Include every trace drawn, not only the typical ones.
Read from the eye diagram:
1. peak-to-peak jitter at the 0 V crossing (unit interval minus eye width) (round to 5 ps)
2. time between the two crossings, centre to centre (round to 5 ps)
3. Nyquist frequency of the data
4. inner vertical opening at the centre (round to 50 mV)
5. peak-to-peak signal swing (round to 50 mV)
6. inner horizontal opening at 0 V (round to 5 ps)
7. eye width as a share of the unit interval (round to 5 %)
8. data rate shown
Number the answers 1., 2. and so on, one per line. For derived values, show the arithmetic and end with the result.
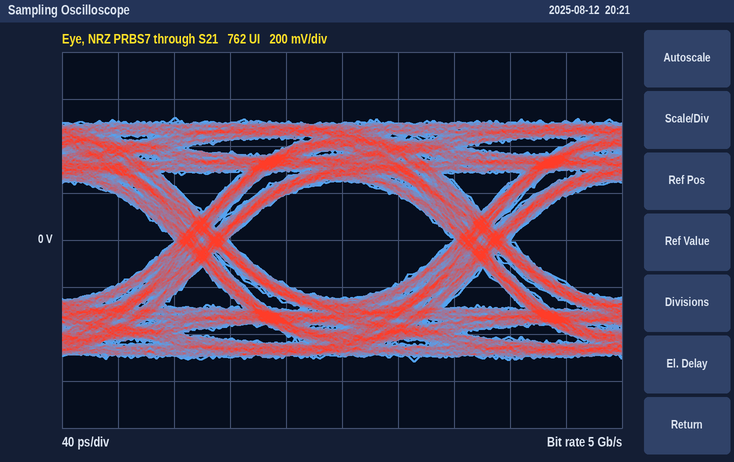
1. 40 ps
2. 200 ps
3. 2.5 GHz
4. 500 mV
5. 1.05 V
6. 160 ps
7. 160 ps / 200 ps ≈ 80 %
8. 5 Gb/s
